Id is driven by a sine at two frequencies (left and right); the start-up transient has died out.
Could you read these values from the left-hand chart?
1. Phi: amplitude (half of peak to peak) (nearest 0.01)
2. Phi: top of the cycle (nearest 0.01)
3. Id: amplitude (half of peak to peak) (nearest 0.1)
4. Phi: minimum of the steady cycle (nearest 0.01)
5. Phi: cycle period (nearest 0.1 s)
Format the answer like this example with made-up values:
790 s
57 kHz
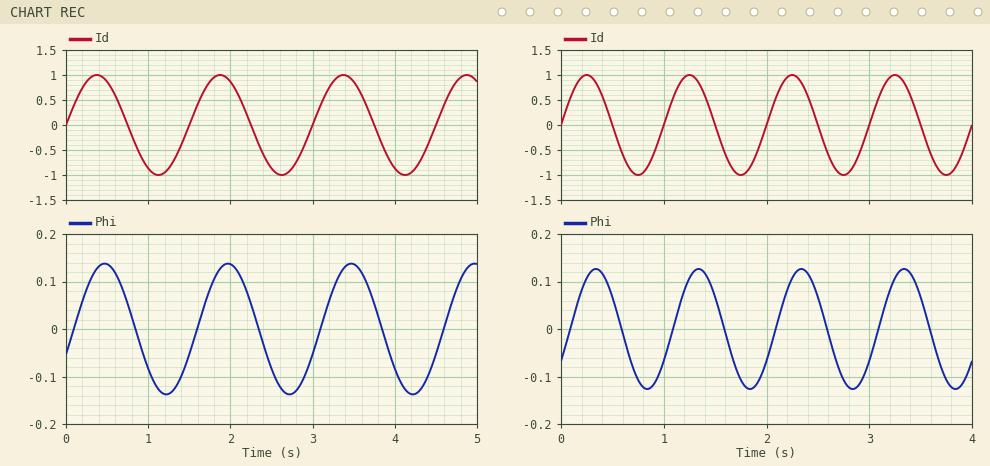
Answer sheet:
0.14
0.14
1.0
-0.14
1.5 s
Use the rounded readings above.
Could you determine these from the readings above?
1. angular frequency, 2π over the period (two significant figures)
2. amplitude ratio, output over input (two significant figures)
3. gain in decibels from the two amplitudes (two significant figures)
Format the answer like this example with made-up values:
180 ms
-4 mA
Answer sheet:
4.2 rad/s
0.14
-17 dB
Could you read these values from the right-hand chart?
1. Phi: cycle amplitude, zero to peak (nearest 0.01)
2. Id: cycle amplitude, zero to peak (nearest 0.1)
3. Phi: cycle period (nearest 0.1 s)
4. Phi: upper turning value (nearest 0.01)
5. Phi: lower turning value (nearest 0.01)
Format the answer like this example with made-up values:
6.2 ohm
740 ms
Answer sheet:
0.13
1.0
1.0 s
0.13
-0.13
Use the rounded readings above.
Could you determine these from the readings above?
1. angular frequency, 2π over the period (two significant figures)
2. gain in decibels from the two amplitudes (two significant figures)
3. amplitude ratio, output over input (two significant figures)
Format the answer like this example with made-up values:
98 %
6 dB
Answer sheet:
6.3 rad/s
-18 dB
0.13
